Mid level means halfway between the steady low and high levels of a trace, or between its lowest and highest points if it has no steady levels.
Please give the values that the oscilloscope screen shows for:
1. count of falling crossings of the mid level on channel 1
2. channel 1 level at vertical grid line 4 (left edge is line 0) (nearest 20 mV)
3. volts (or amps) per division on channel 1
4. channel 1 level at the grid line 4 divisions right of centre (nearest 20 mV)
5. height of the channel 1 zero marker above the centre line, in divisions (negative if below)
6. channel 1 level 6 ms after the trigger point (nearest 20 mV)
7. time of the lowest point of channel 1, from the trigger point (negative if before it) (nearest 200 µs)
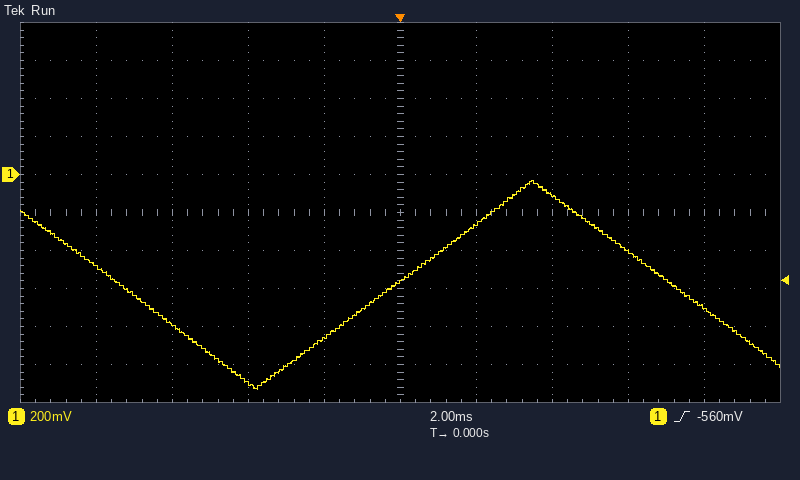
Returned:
2
-860 mV
200 mV
-700 mV
+1.0 div
-400 mV
-3.8 ms
